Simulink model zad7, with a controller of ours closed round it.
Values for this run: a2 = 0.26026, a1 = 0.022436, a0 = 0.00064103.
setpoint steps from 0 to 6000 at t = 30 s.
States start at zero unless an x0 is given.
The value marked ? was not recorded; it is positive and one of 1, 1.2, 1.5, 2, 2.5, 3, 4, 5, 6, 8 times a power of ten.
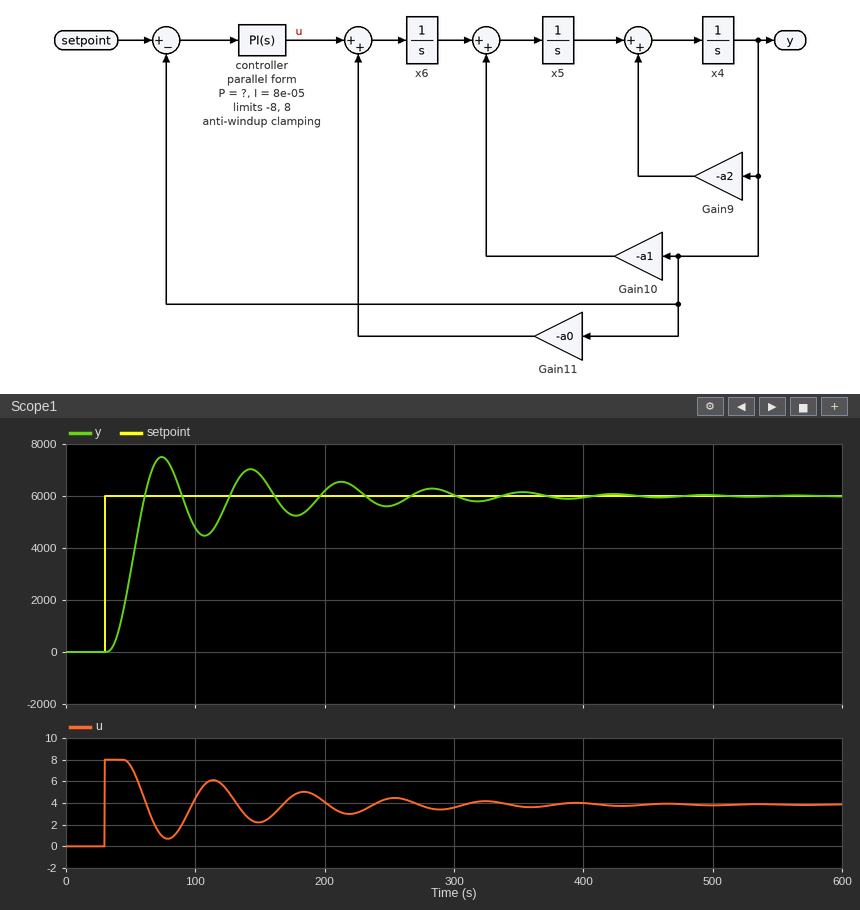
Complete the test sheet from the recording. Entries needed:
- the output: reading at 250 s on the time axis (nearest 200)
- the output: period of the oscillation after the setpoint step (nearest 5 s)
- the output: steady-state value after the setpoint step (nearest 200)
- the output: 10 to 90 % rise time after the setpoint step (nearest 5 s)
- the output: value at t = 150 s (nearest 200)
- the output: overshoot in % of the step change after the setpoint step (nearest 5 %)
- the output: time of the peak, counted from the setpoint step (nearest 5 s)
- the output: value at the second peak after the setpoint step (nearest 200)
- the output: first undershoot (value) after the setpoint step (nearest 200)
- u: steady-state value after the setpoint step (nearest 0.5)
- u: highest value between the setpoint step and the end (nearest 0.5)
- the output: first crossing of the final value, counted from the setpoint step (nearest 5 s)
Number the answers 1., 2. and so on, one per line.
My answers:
1. 5600
2. 70 s
3. 6000
4. 20 s
5. 6800
6. 25 %
7. 45 s
8. 7000
9. 4400
10. 4.0
11. 8.0
12. 30 s
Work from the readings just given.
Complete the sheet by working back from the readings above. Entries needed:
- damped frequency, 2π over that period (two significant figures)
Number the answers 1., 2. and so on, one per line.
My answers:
1. 0.090 rad/s
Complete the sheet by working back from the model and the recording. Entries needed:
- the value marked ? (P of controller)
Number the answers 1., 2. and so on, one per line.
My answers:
1. 0.0015
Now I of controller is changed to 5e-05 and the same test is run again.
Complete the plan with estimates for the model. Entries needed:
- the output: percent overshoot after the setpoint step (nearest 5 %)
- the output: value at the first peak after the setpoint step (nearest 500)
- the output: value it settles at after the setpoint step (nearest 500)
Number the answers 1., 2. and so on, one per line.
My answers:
1. 15 %
2. 7000
3. 6000
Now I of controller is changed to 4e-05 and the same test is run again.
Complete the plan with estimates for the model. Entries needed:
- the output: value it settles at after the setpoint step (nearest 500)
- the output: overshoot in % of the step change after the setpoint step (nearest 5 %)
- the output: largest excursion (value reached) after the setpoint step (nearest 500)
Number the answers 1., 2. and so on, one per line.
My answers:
1. 6000
2. 10 %
3. 6500
